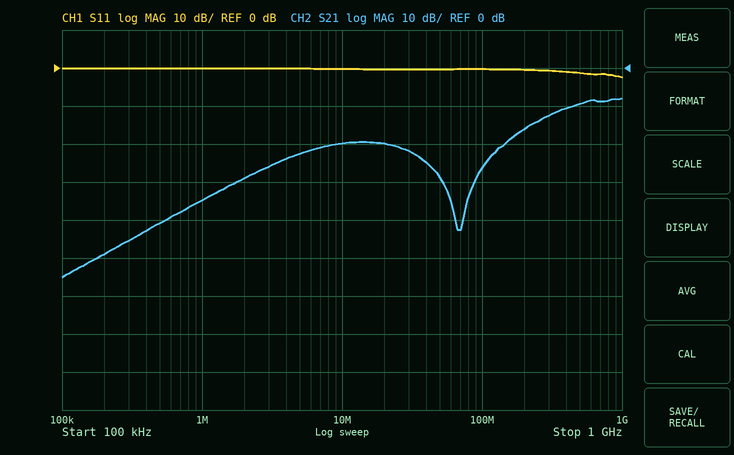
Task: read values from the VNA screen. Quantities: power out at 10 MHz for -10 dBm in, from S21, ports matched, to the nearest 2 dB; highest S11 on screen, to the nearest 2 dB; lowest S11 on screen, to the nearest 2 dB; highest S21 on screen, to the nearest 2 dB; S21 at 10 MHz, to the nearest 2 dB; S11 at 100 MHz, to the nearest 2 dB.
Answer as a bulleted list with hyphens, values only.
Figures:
- -30 dBm
- 0 dB
- -2 dB
- -8 dB
- -20 dB
- 0 dB
